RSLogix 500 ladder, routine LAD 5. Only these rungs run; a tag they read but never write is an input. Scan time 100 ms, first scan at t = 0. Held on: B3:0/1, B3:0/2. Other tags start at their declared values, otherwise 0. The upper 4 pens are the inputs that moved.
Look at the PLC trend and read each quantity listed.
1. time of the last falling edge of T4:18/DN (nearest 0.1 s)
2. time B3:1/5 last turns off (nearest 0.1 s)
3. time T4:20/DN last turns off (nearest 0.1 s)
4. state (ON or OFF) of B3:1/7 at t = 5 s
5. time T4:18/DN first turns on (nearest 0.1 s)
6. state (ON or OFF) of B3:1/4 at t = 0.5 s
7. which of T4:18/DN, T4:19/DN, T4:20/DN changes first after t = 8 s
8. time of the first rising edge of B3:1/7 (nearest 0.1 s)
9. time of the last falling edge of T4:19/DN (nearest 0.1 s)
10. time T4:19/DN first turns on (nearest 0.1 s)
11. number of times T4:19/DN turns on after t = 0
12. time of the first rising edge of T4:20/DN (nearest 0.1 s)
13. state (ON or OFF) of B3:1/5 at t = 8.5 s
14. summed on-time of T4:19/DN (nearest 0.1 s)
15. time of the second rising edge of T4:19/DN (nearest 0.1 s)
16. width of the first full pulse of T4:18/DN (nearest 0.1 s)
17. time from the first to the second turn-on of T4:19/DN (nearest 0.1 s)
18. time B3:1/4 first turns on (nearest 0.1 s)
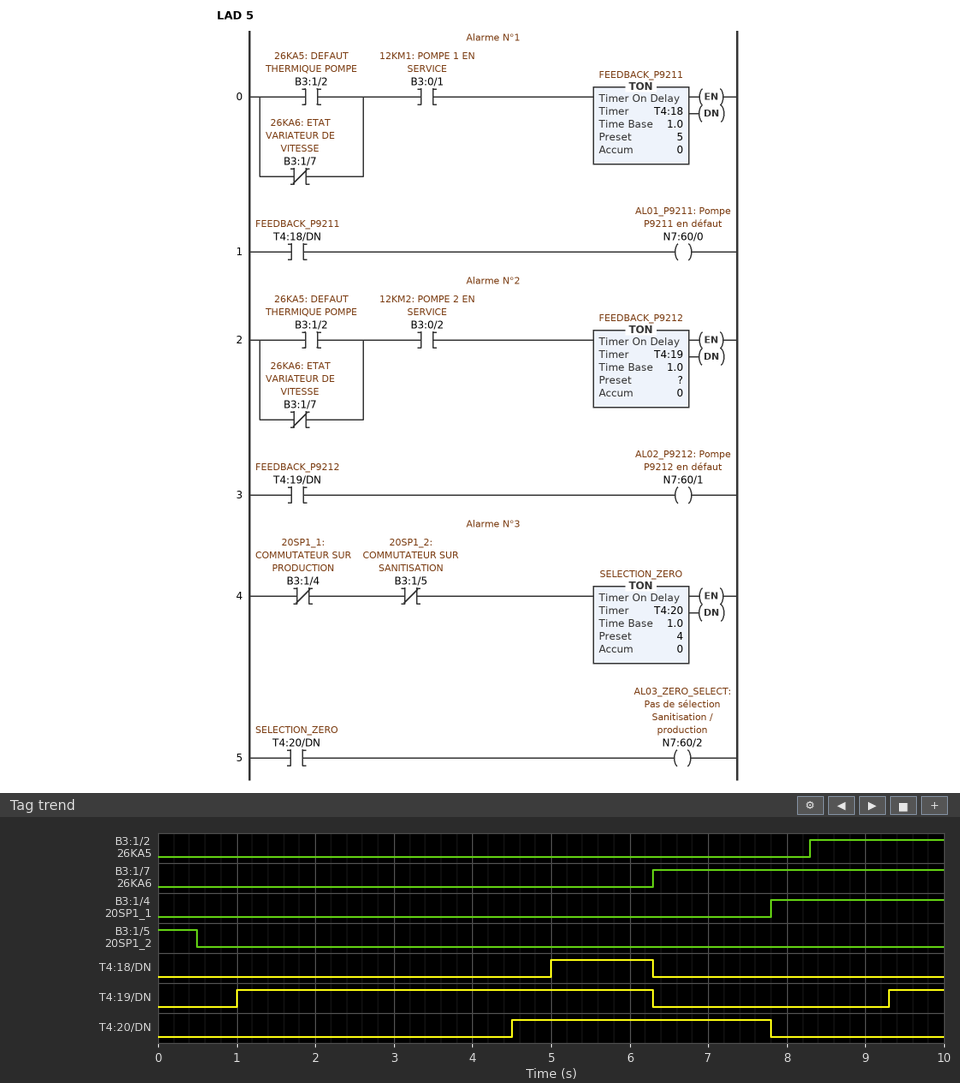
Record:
6.3 s
0.5 s
7.8 s
OFF
5.0 s
OFF
T4:19/DN
6.3 s
6.3 s
1.0 s
2
4.5 s
OFF
6.0 s
9.3 s
1.3 s
8.3 s
7.8 s
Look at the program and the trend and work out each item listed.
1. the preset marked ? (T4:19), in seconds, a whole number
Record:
1 s
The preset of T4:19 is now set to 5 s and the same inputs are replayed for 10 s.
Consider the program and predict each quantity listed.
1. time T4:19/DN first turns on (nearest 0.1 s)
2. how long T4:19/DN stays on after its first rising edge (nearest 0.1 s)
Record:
5.0 s
1.3 s
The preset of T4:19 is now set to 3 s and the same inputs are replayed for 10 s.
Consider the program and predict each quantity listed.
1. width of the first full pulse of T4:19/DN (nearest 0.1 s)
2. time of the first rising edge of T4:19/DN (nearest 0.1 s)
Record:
3.3 s
3.0 s
